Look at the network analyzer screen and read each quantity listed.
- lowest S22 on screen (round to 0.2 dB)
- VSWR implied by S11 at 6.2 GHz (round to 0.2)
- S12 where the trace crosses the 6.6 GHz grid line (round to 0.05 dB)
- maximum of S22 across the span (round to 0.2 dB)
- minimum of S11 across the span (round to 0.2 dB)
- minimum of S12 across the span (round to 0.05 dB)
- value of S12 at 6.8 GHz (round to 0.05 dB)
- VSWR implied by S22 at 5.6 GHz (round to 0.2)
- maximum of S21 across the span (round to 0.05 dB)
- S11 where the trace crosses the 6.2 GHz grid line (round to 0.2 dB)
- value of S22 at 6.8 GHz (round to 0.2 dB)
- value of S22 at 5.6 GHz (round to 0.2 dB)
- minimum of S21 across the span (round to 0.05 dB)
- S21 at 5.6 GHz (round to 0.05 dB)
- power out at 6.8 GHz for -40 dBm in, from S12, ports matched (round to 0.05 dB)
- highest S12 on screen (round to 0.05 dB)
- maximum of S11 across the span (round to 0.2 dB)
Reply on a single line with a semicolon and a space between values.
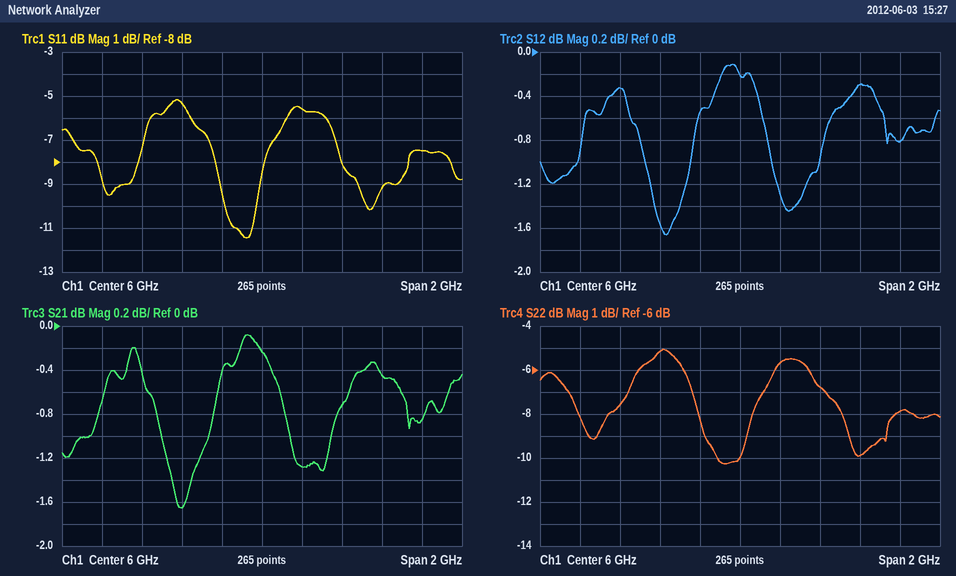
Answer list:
-10.2 dB; 3.2; -0.30 dB; -5.0 dB; -11.4 dB; -1.65 dB; -0.80 dB; 3.4; -0.10 dB; -5.6 dB; -7.8 dB; -5.2 dB; -1.65 dB; -1.65 dB; -40.80 dBm; -0.10 dB; -5.2 dB
